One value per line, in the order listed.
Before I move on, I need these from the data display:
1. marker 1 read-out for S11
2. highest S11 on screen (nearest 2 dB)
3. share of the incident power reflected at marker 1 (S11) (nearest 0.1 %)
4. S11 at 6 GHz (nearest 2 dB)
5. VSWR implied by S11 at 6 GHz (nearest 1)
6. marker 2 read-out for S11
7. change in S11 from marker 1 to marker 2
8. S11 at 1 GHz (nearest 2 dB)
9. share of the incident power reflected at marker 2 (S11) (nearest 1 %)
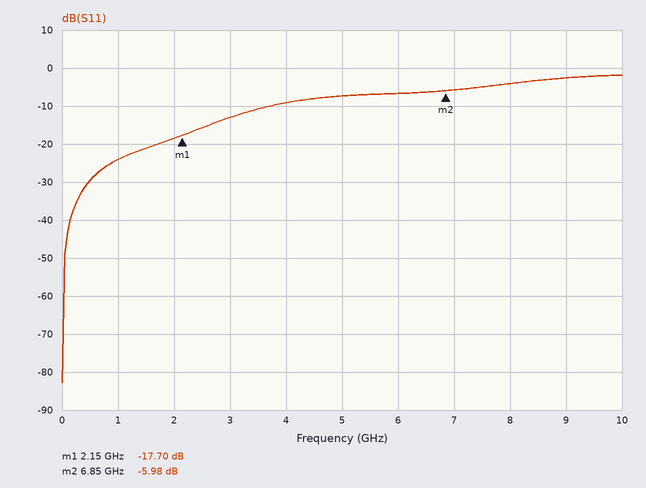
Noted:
-17.70 dB
-2 dB
1.7 %
-6 dB
3
-5.98 dB
11.72 dB
-24 dB
25 %
